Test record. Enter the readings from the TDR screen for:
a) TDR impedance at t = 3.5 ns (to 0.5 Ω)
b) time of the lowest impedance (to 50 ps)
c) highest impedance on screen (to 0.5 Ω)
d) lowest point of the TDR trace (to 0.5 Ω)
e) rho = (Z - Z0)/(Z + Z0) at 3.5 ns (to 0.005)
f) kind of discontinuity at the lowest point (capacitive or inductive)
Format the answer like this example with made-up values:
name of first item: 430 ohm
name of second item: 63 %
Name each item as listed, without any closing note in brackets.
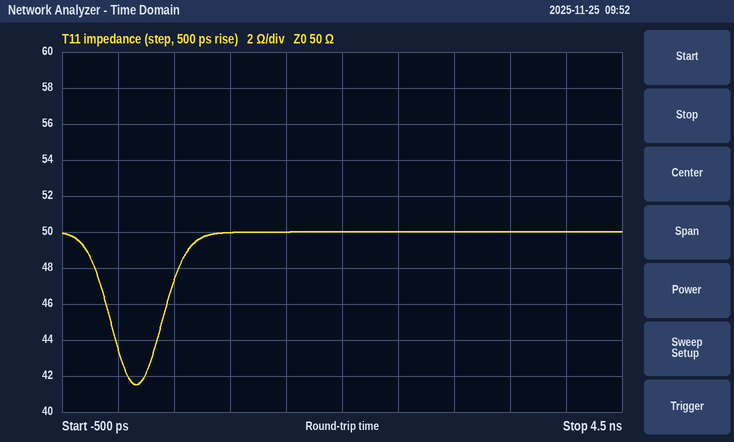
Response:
TDR impedance at t = 3.5 ns: 50.0 Ω
time of the lowest impedance: 150 ps
highest impedance on screen: 50.0 Ω
lowest point of the TDR trace: 41.5 Ω
rho = (Z - Z0)/(Z + Z0) at 3.5 ns: 0.000
kind of discontinuity at the lowest point: capacitive
